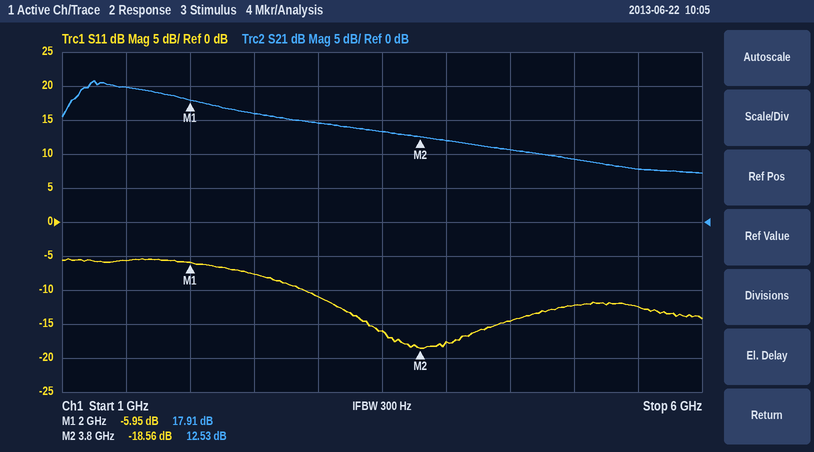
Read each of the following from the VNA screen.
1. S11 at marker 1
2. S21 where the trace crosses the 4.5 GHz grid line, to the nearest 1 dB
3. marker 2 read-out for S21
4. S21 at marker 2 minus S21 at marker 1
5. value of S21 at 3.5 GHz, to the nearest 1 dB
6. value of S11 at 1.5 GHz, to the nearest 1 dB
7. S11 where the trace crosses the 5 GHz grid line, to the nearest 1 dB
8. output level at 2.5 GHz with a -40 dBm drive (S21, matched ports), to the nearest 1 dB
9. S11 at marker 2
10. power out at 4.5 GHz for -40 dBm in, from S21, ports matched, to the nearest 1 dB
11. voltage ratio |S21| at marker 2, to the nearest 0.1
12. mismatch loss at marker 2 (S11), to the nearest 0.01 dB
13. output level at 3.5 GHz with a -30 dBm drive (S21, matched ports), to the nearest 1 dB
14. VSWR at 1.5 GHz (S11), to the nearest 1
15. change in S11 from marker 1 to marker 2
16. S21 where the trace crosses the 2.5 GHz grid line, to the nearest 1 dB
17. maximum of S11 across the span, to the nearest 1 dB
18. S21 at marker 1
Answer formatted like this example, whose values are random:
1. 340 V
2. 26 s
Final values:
1. -5.95 dB
2. 11 dB
3. 12.53 dB
4. -5.38 dB
5. 13 dB
6. -6 dB
7. -12 dB
8. -24 dBm
9. -18.56 dB
10. -29 dBm
11. 4.2
12. 0.06 dB
13. -17 dBm
14. 3
15. -12.61 dB
16. 16 dB
17. -5 dB
18. 17.91 dB
